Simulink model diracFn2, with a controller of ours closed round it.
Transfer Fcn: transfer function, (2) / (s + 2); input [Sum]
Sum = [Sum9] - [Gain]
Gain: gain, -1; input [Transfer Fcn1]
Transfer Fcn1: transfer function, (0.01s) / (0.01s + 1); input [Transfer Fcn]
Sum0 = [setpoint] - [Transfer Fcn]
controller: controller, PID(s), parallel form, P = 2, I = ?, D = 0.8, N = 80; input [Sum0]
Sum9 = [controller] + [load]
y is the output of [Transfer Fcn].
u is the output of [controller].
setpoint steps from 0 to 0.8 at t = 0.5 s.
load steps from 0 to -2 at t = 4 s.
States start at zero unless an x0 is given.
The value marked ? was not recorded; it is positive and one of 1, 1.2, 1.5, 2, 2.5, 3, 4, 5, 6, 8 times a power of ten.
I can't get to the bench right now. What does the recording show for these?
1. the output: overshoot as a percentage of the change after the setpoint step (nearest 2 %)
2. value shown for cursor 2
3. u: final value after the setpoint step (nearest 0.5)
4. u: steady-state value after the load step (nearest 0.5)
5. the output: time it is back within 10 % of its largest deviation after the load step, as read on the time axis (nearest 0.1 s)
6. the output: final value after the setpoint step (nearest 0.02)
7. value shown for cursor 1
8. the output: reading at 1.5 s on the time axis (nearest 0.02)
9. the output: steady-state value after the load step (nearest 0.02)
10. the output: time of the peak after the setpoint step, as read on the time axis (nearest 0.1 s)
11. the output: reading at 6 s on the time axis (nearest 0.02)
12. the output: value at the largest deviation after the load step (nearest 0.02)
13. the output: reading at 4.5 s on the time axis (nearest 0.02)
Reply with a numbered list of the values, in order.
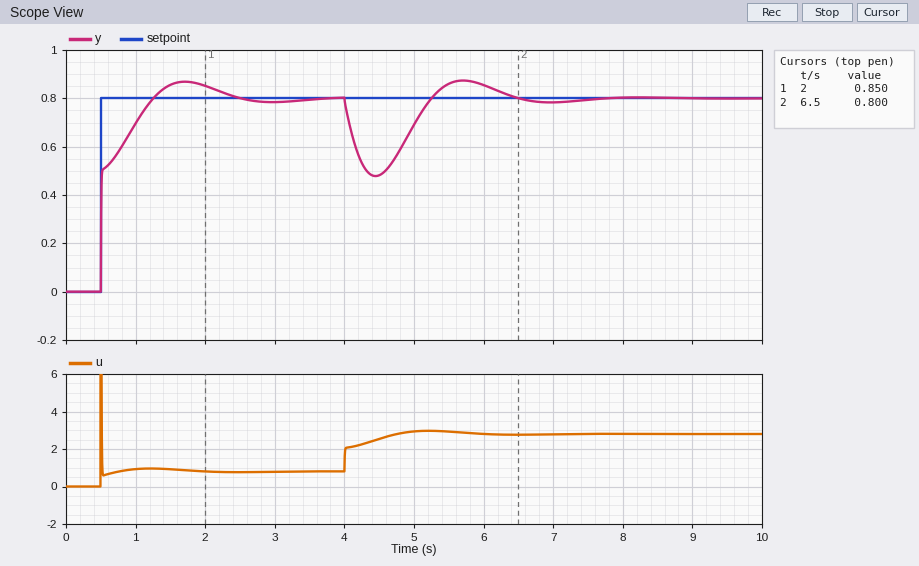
1. 8 %
2. 0.800
3. 1.0
4. 3.0
5. 6.2 s
6. 0.80
7. 0.850
8. 0.86
9. 0.80
10. 1.7 s
11. 0.86
12. 0.48
13. 0.48
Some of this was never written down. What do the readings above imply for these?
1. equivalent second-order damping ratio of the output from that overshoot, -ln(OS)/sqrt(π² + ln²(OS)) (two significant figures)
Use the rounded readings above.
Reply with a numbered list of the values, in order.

1. 0.63
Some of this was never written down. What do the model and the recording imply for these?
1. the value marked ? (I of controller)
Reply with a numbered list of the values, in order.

1. 10
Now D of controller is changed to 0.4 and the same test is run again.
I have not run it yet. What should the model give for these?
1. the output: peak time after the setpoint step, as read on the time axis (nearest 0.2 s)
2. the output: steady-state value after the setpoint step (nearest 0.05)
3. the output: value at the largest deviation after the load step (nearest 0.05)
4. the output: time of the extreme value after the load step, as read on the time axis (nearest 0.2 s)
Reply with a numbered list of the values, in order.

1. 1.4 s
2. 0.80
3. 0.45
4. 4.4 s
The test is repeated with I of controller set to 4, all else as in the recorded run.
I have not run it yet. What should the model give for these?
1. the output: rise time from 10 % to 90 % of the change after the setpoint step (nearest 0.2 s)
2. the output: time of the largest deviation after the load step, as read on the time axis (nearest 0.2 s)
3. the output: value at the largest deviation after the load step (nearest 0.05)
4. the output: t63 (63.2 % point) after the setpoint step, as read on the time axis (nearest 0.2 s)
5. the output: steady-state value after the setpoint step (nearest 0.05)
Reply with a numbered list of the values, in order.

1. 1.0 s
2. 4.6 s
3. 0.40
4. 0.6 s
5. 0.80
